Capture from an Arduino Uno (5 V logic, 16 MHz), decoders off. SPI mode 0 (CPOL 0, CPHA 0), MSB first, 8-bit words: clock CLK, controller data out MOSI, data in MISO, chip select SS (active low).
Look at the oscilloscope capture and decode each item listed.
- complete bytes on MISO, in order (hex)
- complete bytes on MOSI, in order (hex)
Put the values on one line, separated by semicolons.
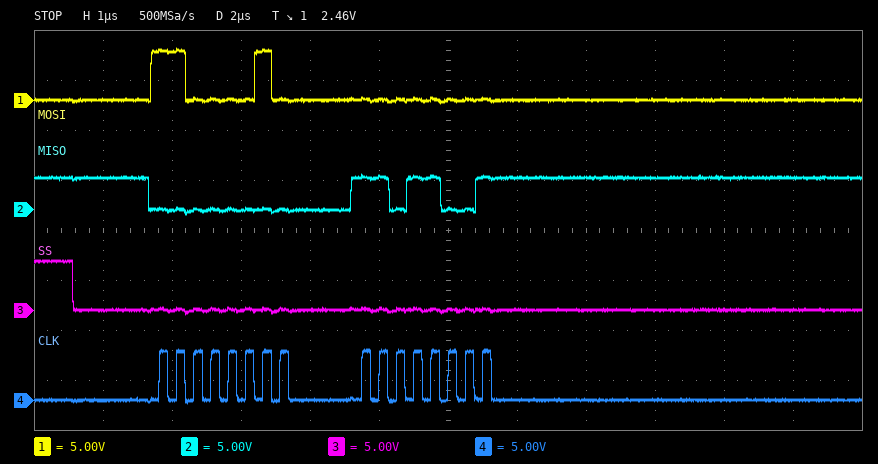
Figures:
00 D9; C2 00
